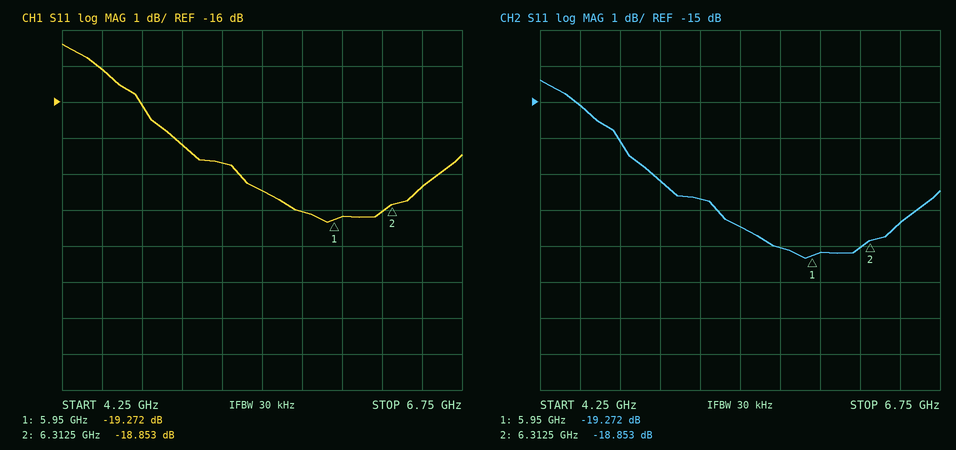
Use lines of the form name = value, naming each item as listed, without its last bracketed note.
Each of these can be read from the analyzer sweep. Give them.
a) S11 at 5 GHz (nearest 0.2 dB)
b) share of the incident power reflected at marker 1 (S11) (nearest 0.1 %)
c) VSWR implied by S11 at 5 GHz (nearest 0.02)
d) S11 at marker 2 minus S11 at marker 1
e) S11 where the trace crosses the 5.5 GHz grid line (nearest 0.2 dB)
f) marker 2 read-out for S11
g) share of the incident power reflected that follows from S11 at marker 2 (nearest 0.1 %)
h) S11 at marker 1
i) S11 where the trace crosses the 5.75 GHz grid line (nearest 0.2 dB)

S11 at 5 GHz = -17.2 dB
share of the incident power reflected at marker 1 (S11) = 1.2 %
VSWR implied by S11 at 5 GHz = 1.32
S11 at marker 2 minus S11 at marker 1 = 0.419 dB
S11 where the trace crosses the 5.5 GHz grid line = -18.4 dB
marker 2 read-out for S11 = -18.853 dB
share of the incident power reflected that follows from S11 at marker 2 = 1.3 %
S11 at marker 1 = -19.272 dB
S11 where the trace crosses the 5.75 GHz grid line = -19.0 dB
